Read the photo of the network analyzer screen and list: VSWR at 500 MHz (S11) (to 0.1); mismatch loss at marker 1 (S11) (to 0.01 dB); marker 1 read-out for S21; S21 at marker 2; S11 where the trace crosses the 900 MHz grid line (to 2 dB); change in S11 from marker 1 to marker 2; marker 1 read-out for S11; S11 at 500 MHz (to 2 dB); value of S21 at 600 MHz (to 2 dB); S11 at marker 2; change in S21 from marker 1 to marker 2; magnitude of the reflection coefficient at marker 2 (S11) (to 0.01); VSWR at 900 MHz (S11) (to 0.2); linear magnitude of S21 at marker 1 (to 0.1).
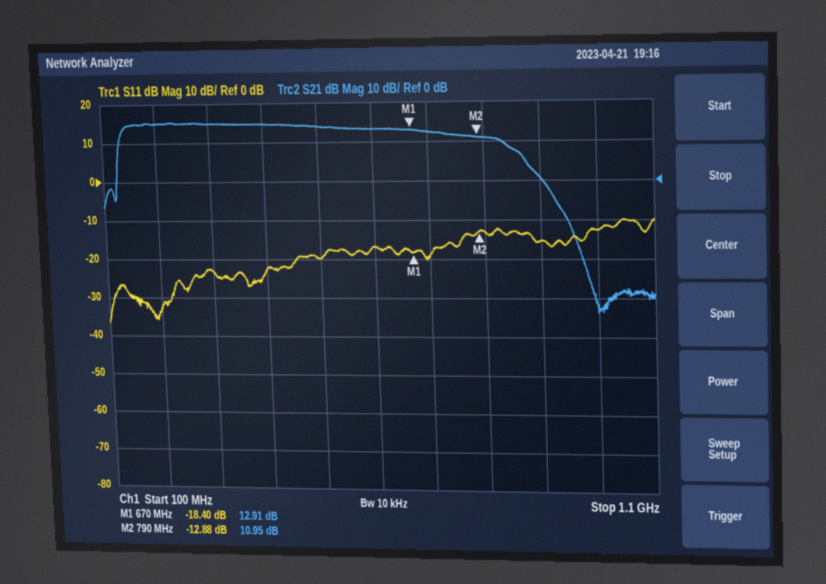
1.2
0.06 dB
12.91 dB
10.95 dB
-16 dB
5.52 dB
-18.40 dB
-20 dB
14 dB
-12.88 dB
-1.96 dB
0.23
1.4
4.4
